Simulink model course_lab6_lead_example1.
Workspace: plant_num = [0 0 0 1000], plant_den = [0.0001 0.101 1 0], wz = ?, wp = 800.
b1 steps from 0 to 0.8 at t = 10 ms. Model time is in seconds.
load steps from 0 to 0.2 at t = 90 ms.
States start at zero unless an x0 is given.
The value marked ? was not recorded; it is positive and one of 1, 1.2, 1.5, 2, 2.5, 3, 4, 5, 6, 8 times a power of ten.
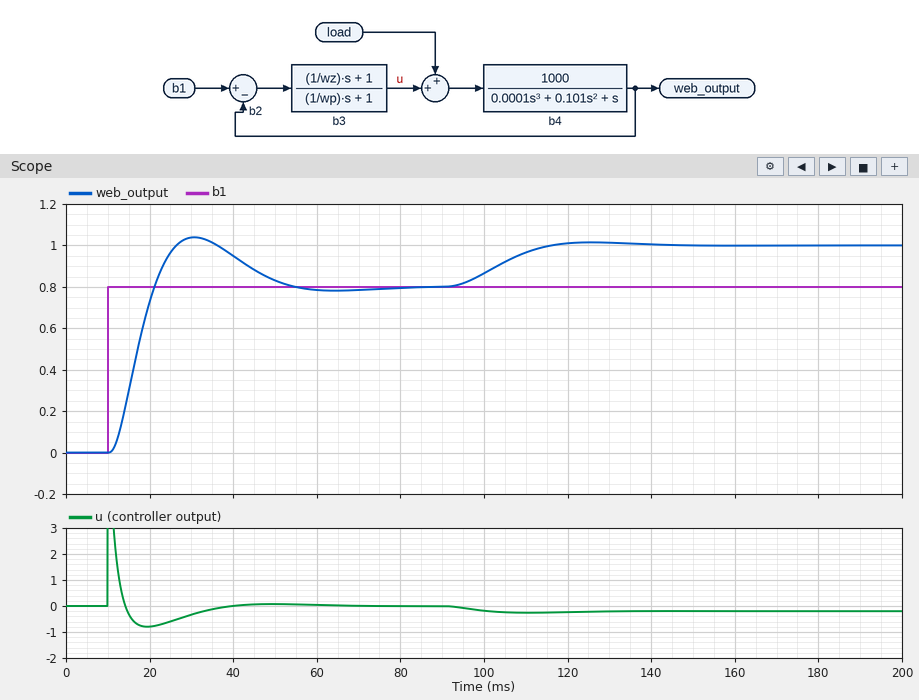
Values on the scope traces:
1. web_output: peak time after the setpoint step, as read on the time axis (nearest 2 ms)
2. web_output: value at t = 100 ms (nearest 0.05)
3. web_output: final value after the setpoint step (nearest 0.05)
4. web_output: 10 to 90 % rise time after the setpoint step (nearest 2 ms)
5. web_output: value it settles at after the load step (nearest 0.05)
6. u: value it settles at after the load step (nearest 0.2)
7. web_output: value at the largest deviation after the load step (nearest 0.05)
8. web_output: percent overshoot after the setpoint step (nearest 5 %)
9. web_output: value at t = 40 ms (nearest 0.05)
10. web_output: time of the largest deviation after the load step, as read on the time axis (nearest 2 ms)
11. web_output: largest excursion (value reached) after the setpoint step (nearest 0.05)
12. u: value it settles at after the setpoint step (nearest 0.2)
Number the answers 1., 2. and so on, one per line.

1. 30 ms
2. 0.85
3. 0.80
4. 8 ms
5. 1.00
6. -0.2
7. 1.00
8. 30 %
9. 0.95
10. 126 ms
11. 1.05
12. 0.0
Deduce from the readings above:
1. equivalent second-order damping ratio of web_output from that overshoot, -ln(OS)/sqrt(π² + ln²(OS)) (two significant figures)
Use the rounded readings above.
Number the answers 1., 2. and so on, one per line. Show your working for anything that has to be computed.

1. ln(0.3) = -1.204; 1.204 / sqrt(9.870 + 1.450) = 0.36
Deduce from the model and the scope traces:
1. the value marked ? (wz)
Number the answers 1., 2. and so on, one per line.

1. 80
